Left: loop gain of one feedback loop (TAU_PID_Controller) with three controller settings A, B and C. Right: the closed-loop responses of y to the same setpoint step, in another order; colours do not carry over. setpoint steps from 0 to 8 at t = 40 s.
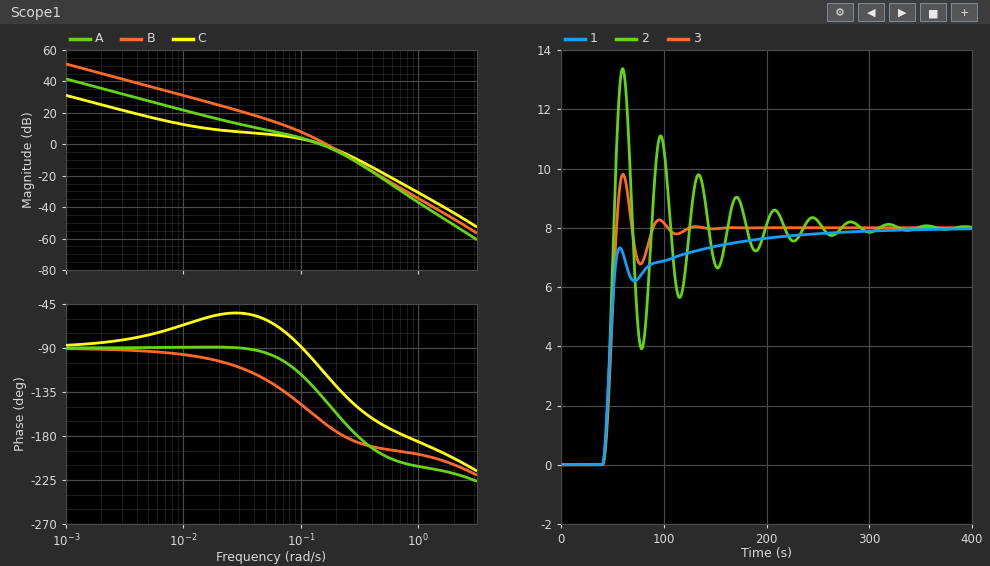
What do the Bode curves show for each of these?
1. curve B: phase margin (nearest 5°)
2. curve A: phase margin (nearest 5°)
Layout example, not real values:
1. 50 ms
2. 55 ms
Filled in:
1. 10°
2. 40°
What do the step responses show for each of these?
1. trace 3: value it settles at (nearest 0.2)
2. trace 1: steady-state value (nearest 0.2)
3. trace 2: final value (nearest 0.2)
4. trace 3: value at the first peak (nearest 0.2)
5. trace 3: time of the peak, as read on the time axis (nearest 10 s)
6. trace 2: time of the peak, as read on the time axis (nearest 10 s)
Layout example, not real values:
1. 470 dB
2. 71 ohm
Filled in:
1. 8.0
2. 8.0
3. 8.0
4. 9.8
5. 60 s
6. 60 s
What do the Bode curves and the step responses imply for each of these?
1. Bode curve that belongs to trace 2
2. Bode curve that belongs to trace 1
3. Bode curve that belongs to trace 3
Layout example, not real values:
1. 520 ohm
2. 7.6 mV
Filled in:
1. B
2. C
3. A
